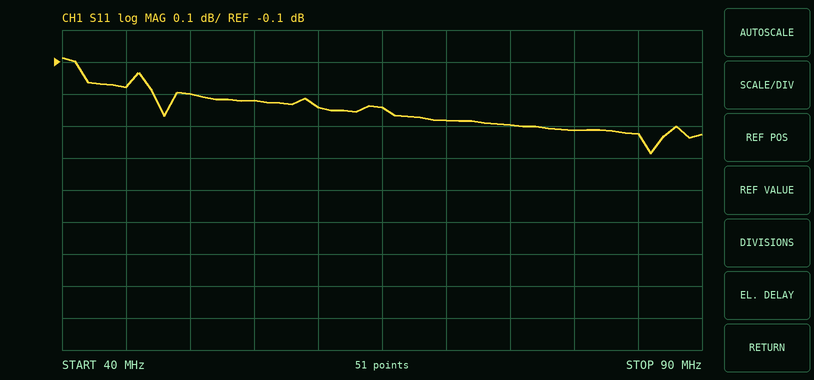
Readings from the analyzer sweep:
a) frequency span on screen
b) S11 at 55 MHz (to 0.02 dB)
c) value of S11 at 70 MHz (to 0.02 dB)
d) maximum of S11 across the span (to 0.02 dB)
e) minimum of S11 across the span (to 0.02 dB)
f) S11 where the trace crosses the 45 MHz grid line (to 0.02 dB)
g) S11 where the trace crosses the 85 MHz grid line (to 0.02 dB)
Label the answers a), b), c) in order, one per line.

a) 50 MHz
b) -0.22 dB
c) -0.28 dB
d) -0.08 dB
e) -0.38 dB
f) -0.18 dB
g) -0.32 dB
